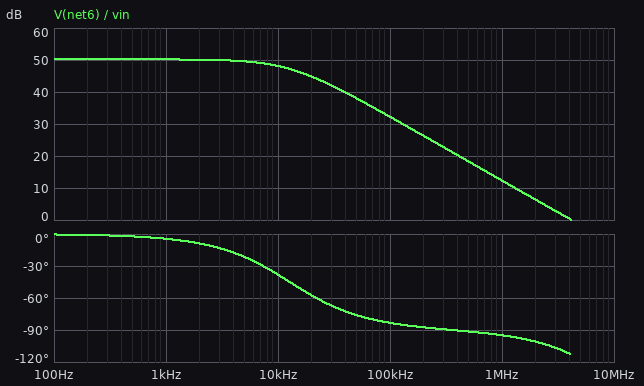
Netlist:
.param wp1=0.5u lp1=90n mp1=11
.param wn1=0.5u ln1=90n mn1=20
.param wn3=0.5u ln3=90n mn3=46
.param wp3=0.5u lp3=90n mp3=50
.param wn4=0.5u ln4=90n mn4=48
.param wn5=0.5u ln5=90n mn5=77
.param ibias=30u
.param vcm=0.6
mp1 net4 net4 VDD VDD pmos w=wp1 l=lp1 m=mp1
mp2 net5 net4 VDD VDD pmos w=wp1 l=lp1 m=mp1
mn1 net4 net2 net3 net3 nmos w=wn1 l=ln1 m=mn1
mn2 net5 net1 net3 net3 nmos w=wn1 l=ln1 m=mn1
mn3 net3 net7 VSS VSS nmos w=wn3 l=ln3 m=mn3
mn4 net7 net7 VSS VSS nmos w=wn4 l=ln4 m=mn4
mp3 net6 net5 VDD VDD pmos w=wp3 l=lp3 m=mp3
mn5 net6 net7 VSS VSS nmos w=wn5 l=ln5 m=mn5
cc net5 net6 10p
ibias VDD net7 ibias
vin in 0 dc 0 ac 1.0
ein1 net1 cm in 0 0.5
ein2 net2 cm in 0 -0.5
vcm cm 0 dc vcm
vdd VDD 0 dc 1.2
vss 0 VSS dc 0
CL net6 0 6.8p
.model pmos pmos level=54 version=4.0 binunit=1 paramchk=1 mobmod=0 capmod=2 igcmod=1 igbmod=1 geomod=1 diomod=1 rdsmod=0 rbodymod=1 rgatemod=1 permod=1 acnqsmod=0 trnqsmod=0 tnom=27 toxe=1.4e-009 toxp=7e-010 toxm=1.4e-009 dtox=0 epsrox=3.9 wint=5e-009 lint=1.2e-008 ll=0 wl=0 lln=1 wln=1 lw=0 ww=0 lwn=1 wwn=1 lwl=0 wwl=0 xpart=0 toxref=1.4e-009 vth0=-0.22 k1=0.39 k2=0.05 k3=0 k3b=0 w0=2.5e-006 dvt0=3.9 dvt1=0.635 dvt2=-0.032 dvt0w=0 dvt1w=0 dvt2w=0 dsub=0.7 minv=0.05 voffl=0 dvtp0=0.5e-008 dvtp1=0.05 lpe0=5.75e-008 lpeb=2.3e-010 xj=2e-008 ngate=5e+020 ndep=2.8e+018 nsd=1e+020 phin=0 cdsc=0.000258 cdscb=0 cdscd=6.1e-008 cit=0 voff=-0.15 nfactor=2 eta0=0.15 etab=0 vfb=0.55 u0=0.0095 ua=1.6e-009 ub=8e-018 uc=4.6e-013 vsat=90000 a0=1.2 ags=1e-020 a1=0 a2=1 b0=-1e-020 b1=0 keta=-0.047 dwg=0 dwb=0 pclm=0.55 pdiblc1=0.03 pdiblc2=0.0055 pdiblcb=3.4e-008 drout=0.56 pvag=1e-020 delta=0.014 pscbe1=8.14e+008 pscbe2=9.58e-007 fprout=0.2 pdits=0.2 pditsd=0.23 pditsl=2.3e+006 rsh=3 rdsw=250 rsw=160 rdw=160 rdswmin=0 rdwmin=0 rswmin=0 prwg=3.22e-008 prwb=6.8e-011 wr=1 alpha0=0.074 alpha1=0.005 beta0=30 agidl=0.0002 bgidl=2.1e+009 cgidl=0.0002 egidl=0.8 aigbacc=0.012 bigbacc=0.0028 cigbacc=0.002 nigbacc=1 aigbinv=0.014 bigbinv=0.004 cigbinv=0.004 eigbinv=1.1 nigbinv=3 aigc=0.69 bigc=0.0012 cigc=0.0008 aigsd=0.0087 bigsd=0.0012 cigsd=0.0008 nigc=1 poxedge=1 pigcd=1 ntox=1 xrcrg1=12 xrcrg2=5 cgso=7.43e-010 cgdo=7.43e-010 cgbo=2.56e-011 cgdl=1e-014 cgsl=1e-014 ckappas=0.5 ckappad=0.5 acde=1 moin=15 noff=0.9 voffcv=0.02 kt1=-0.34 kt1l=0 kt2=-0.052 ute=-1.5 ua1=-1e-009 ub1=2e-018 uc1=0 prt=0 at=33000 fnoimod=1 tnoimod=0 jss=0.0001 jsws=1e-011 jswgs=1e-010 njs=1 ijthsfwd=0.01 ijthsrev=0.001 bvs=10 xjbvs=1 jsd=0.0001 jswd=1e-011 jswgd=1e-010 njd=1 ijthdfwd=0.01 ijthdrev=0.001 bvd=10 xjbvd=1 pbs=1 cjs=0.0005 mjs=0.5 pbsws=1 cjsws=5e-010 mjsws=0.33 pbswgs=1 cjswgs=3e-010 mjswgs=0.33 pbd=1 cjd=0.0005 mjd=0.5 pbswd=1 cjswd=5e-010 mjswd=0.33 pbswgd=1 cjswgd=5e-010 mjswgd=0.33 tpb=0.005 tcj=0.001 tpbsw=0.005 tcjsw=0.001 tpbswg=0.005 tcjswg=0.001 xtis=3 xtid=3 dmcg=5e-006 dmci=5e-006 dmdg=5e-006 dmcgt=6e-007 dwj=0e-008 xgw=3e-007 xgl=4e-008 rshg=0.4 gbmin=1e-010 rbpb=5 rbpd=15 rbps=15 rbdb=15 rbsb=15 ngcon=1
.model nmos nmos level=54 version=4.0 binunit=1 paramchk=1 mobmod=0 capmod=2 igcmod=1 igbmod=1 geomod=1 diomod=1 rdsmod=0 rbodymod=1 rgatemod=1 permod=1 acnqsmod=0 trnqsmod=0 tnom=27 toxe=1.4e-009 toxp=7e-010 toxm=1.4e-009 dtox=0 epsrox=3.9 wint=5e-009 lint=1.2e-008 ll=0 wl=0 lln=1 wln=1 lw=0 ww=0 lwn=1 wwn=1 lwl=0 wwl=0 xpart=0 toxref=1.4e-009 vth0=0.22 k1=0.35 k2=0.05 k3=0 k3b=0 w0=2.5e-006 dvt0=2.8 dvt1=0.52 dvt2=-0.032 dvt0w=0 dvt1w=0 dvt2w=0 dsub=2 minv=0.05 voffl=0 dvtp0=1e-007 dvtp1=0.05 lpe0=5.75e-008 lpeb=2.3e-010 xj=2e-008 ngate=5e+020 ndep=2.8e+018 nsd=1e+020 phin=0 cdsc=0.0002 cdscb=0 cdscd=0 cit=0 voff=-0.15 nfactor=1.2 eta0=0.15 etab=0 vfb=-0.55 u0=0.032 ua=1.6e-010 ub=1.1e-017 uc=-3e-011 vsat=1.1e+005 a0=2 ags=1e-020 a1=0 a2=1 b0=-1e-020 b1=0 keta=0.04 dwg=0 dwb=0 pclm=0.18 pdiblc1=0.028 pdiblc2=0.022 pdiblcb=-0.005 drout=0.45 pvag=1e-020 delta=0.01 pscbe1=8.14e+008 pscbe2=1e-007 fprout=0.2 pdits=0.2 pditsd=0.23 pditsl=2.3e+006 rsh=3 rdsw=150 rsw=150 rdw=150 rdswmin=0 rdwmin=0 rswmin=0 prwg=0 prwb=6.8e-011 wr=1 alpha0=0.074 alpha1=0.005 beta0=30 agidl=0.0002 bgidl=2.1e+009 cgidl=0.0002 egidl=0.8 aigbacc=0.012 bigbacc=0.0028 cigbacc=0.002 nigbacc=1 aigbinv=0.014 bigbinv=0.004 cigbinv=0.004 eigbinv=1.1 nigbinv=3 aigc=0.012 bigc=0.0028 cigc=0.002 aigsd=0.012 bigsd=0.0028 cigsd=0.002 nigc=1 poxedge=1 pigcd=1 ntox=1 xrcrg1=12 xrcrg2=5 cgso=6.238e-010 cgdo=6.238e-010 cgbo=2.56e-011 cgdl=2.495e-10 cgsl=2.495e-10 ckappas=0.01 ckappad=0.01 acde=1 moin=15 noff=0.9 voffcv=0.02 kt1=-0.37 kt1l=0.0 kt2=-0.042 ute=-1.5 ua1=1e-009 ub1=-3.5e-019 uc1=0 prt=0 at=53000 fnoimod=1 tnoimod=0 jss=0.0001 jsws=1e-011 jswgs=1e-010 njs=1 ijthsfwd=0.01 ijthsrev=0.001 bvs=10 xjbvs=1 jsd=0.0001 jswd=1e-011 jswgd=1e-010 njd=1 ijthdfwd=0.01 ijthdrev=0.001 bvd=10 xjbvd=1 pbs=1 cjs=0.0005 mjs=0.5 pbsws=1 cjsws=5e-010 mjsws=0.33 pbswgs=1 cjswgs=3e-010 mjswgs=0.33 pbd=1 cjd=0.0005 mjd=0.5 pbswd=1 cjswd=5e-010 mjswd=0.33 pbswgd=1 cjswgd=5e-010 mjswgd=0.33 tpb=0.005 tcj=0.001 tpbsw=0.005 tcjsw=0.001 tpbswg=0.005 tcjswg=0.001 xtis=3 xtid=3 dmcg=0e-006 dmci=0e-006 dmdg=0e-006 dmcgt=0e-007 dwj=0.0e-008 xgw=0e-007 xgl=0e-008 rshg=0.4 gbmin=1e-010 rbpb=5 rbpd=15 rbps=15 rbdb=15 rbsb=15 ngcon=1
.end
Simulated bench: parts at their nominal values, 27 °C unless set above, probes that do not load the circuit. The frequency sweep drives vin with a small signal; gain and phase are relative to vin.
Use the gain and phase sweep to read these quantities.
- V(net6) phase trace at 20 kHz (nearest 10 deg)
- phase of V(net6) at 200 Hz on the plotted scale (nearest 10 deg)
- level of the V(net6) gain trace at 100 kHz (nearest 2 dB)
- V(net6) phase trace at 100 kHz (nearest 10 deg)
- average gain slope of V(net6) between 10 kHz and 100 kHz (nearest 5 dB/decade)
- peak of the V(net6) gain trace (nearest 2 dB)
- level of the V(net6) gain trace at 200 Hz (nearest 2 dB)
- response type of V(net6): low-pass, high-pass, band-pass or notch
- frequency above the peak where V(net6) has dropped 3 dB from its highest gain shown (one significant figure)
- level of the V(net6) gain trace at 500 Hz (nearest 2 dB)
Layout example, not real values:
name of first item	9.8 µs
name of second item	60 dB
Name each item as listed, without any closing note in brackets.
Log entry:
V(net6) phase trace at 20 kHz	-60 deg
phase of V(net6) at 200 Hz on the plotted scale	0 deg
level of the V(net6) gain trace at 100 kHz	32 dB
V(net6) phase trace at 100 kHz	-80 deg
average gain slope of V(net6) between 10 kHz and 100 kHz	-15 dB/decade
peak of the V(net6) gain trace	50 dB
level of the V(net6) gain trace at 200 Hz	50 dB
response type of V(net6): low-pass, high-pass, band-pass or notch	low-pass
frequency above the peak where V(net6) has dropped 3 dB from its highest gain shown	10 kHz
level of the V(net6) gain trace at 500 Hz	50 dB
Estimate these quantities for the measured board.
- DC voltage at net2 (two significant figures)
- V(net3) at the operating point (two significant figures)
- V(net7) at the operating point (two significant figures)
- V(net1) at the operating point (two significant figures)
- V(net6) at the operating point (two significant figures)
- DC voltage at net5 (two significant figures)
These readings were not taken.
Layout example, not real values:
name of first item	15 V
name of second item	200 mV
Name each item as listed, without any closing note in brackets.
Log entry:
DC voltage at net2	600 mV
V(net3) at the operating point	300 mV
V(net7) at the operating point	300 mV
V(net1) at the operating point	600 mV
V(net6) at the operating point	760 mV
DC voltage at net5	830 mV
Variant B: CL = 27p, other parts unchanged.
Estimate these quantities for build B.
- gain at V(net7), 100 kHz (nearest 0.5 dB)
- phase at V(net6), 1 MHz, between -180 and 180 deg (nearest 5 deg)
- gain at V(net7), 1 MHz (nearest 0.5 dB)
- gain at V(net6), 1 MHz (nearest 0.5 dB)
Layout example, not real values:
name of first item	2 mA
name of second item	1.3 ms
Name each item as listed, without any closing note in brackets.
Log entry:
gain at V(net7), 100 kHz	-15.0 dB
phase at V(net6), 1 MHz, between -180 and 180 deg	-100 deg
gain at V(net7), 1 MHz	-35.0 dB
gain at V(net6), 1 MHz	12.0 dB
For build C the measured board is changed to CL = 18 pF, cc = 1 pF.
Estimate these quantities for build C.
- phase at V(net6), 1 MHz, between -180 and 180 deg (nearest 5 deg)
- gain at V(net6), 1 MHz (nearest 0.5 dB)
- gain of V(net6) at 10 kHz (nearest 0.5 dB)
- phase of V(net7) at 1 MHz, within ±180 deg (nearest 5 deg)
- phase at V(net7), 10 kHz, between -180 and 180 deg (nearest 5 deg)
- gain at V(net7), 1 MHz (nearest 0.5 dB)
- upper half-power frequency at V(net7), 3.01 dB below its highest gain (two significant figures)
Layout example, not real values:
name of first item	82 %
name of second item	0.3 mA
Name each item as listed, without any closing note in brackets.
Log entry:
phase at V(net6), 1 MHz, between -180 and 180 deg	-90 deg
gain at V(net6), 1 MHz	30.5 dB
gain of V(net6) at 10 kHz	50.0 dB
phase of V(net7) at 1 MHz, within ±180 deg	-85 deg
phase at V(net7), 10 kHz, between -180 and 180 deg	-5 deg
gain at V(net7), 1 MHz	-16.5 dB
upper half-power frequency at V(net7), 3.01 dB below its highest gain	100 kHz
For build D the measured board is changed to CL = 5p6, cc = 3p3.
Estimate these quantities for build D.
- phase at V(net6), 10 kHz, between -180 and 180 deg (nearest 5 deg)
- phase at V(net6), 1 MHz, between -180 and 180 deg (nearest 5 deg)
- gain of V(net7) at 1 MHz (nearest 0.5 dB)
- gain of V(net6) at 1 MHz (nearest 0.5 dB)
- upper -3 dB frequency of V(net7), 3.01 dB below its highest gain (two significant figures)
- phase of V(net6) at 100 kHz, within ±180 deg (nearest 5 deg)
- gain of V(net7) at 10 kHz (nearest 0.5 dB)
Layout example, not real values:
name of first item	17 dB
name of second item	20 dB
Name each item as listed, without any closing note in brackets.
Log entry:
phase at V(net6), 10 kHz, between -180 and 180 deg	-15 deg
phase at V(net6), 1 MHz, between -180 and 180 deg	-90 deg
gain of V(net7) at 1 MHz	-25.0 dB
gain of V(net6) at 1 MHz	22.0 dB
upper -3 dB frequency of V(net7), 3.01 dB below its highest gain	38 kHz
phase of V(net6) at 100 kHz, within ±180 deg	-70 deg
gain of V(net7) at 10 kHz	3.0 dB
